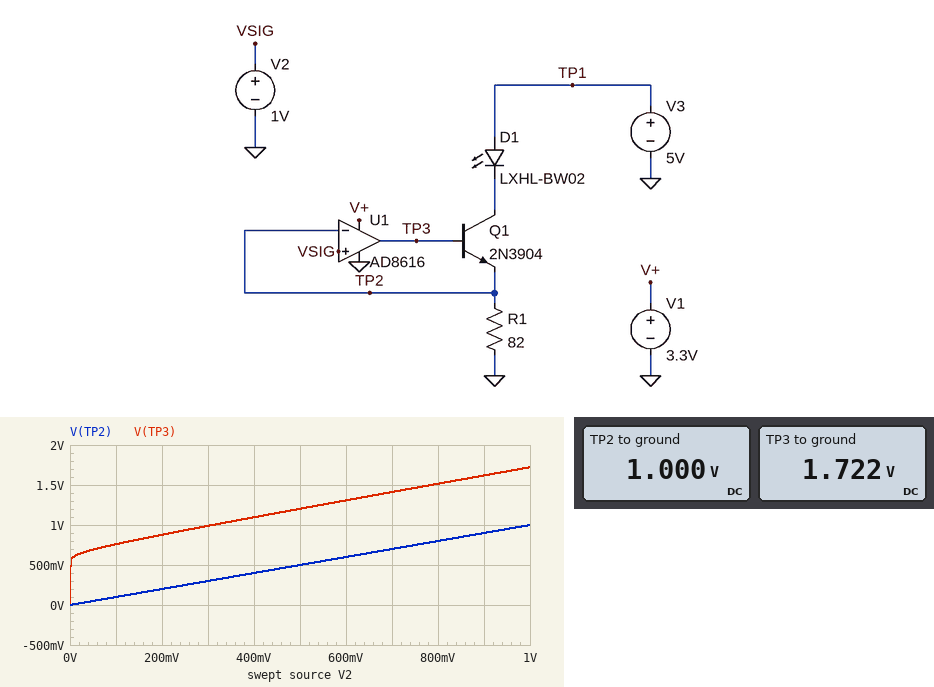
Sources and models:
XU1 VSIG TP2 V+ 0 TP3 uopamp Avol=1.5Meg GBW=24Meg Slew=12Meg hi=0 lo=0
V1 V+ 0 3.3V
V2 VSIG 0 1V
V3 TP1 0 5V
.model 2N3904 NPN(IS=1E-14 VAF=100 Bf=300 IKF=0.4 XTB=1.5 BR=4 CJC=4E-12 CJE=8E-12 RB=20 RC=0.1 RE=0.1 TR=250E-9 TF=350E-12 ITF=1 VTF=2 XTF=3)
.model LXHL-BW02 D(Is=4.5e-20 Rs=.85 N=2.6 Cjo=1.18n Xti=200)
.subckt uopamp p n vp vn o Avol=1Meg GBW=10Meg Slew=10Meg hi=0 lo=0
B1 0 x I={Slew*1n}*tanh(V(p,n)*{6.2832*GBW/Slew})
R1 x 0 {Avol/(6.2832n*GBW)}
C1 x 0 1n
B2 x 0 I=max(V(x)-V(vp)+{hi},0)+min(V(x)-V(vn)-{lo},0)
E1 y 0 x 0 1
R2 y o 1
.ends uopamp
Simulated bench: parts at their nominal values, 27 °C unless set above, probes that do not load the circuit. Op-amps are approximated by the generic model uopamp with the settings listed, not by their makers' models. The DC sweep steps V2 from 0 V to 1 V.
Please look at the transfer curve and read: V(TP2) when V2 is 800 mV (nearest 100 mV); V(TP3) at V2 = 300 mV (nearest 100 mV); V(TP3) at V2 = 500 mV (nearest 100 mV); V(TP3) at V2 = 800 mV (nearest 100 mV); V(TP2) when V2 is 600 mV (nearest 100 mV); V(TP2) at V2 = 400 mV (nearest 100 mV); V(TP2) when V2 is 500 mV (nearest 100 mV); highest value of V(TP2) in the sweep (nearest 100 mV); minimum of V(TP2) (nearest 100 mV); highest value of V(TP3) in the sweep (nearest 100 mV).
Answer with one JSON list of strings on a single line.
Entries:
["800 mV", "1.0 V", "1.2 V", "1.5 V", "600 mV", "400 mV", "500 mV", "1.0 V", "0 V", "1.7 V"]
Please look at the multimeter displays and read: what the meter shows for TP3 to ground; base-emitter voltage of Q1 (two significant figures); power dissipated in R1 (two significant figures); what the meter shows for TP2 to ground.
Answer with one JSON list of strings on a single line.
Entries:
["1.722 V", "720 mV", "12 mW", "1.000 V"]
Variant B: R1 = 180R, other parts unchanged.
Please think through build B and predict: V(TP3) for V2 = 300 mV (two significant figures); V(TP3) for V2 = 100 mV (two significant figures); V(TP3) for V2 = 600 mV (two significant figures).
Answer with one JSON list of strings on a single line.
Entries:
["970 mV", "740 mV", "1.3 V"]
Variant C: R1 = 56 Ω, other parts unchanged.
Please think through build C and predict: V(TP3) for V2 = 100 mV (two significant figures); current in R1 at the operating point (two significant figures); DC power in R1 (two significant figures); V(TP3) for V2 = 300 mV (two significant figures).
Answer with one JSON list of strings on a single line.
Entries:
["770 mV", "18 mA", "18 mW", "1.0 V"]
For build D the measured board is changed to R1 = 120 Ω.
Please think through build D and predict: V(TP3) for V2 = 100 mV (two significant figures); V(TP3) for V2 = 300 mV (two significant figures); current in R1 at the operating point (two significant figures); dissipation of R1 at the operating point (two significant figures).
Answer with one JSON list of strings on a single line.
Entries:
["750 mV", "980 mV", "8.3 mA", "8.3 mW"]
